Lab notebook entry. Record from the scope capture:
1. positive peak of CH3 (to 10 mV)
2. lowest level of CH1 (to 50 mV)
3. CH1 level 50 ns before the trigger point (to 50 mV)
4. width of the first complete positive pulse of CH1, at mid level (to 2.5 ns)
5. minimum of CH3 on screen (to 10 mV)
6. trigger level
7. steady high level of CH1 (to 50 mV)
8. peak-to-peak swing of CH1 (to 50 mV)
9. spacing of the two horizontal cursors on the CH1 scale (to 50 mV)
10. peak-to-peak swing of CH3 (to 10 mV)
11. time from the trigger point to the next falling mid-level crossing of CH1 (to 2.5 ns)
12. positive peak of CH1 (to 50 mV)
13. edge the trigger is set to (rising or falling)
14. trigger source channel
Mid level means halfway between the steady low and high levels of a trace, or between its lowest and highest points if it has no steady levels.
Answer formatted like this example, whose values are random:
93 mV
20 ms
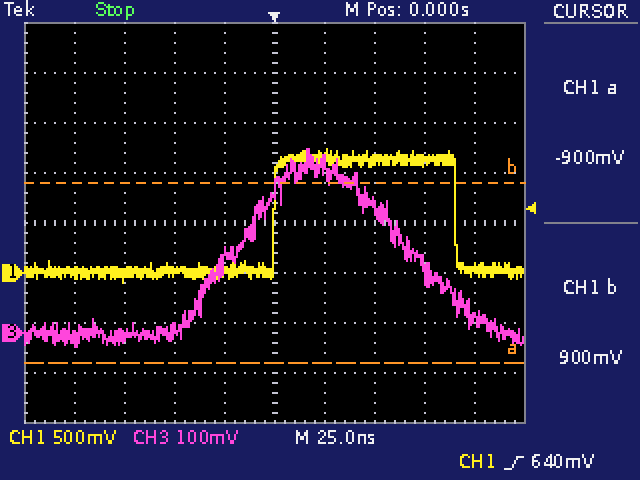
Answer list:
370 mV
-100 mV
0 mV
90.0 ns
-30 mV
640 mV
1.15 V
1.35 V
1.80 V
400 mV
90.0 ns
1.25 V
rising
CH1
